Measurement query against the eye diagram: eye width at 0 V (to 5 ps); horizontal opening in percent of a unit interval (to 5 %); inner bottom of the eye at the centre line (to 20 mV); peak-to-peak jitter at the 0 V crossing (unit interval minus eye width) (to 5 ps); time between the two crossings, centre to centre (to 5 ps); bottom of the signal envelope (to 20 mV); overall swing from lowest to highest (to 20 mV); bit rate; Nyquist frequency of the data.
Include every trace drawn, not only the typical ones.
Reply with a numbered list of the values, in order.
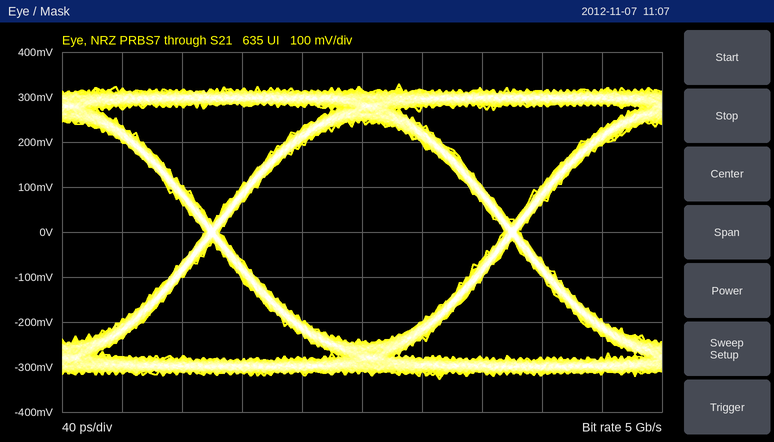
1. 190 ps
2. 95 %
3. -240 mV
4. 10 ps
5. 200 ps
6. -320 mV
7. 660 mV
8. 5 Gb/s
9. 2.5 GHz
